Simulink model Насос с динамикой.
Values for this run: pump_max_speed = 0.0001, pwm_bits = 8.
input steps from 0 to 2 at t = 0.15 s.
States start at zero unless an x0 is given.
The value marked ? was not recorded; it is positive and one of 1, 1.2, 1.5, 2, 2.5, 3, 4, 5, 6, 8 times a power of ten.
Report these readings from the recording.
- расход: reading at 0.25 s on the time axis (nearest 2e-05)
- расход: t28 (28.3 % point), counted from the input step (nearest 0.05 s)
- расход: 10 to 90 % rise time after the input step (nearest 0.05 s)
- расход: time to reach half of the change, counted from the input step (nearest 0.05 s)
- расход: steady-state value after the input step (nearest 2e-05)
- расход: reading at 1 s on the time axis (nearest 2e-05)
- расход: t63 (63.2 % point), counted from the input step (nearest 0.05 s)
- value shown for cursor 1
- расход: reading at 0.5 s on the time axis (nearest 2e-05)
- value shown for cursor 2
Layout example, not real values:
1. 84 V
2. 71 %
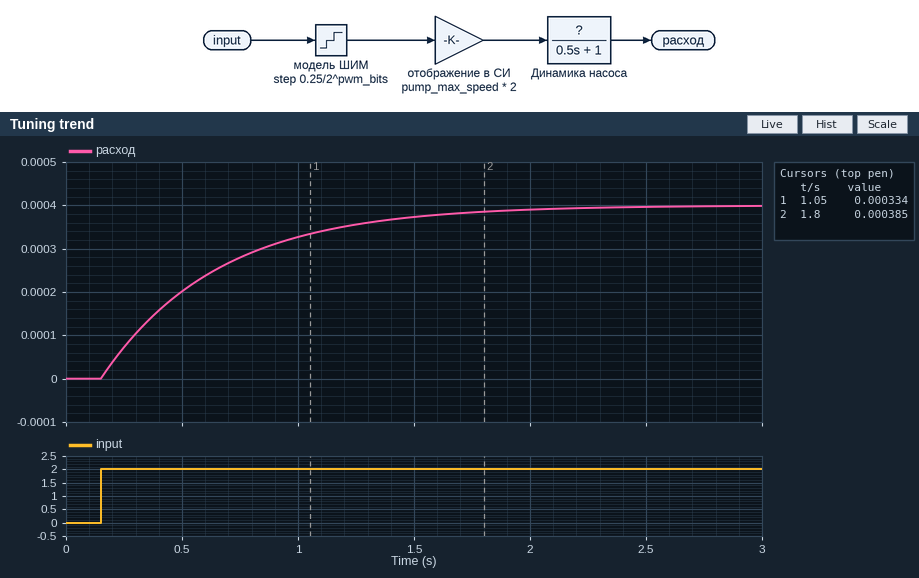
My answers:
1. 0.00008
2. 0.15 s
3. 1.10 s
4. 0.35 s
5. 0.00040
6. 0.00032
7. 0.50 s
8. 0.000334
9. 0.00020
10. 0.000385
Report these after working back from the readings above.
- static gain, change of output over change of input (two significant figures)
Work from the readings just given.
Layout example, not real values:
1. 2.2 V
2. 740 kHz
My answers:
1. 0.00020
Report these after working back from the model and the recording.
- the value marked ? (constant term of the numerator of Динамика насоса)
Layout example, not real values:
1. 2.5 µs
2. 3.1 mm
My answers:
1. 1
